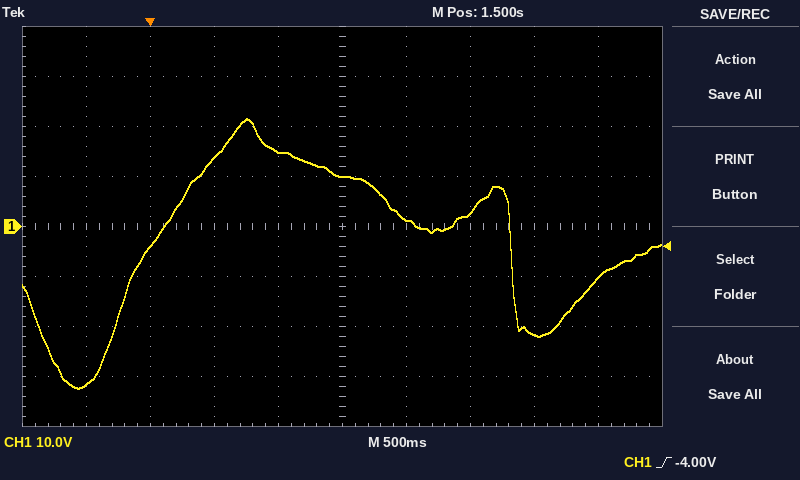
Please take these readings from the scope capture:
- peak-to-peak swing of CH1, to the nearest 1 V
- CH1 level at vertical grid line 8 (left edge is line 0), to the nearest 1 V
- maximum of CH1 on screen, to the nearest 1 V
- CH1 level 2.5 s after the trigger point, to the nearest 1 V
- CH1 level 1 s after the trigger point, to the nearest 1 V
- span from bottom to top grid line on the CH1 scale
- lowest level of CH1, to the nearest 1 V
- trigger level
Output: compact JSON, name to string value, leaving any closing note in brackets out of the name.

{"peak-to-peak swing of CH1, to the nearest 1 V": "54 V", "CH1 level at vertical grid line 8 (left edge is line 0), to the nearest 1 V": "-22 V", "maximum of CH1 on screen, to the nearest 1 V": "22 V", "CH1 level 2.5 s after the trigger point, to the nearest 1 V": "3 V", "CH1 level 1 s after the trigger point, to the nearest 1 V": "15 V", "span from bottom to top grid line on the CH1 scale": "80 V", "lowest level of CH1, to the nearest 1 V": "-32 V", "trigger level": "-4.00 V"}
